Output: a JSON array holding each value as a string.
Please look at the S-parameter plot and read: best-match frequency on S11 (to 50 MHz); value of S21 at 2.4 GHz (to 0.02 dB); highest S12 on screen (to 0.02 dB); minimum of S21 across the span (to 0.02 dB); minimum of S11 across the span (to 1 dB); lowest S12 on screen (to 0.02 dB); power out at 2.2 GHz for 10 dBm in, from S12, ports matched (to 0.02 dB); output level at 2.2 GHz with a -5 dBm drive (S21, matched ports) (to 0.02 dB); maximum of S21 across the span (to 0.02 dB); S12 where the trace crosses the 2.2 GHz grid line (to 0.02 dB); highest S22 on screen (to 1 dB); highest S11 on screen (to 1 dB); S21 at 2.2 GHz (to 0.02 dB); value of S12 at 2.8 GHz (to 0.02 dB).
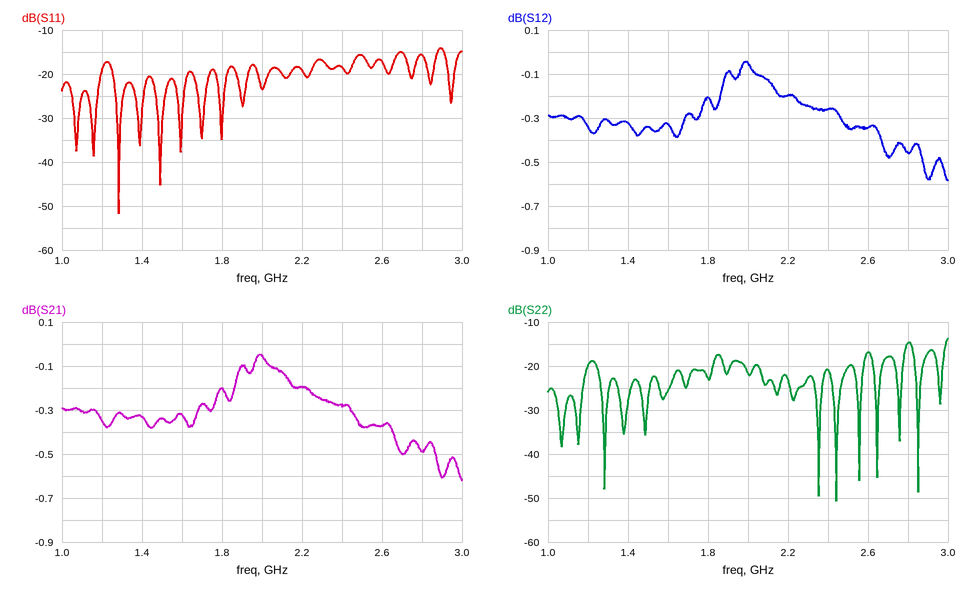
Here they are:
["1.30 GHz", "-0.28 dB", "-0.04 dB", "-0.62 dB", "-52 dB", "-0.58 dB", "9.80 dBm", "-5.20 dBm", "-0.04 dB", "-0.20 dB", "-14 dB", "-14 dB", "-0.20 dB", "-0.46 dB"]
